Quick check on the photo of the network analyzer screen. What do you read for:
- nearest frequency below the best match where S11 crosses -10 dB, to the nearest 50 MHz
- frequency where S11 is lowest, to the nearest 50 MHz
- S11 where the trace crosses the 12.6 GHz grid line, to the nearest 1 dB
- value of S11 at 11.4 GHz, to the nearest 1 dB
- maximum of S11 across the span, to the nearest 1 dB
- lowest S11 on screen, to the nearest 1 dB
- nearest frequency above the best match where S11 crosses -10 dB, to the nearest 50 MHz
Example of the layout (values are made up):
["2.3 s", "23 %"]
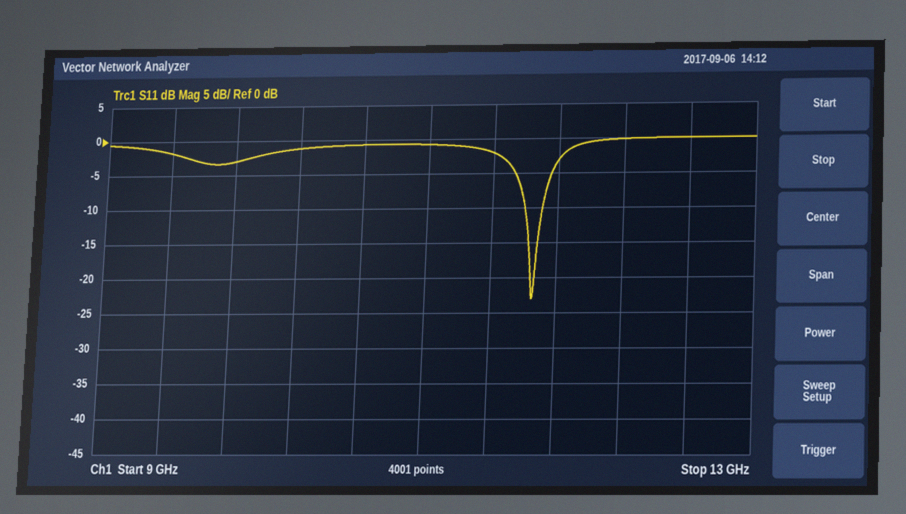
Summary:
["11.60 GHz", "11.65 GHz", "0 dB", "-2 dB", "0 dB", "-23 dB", "11.70 GHz"]
